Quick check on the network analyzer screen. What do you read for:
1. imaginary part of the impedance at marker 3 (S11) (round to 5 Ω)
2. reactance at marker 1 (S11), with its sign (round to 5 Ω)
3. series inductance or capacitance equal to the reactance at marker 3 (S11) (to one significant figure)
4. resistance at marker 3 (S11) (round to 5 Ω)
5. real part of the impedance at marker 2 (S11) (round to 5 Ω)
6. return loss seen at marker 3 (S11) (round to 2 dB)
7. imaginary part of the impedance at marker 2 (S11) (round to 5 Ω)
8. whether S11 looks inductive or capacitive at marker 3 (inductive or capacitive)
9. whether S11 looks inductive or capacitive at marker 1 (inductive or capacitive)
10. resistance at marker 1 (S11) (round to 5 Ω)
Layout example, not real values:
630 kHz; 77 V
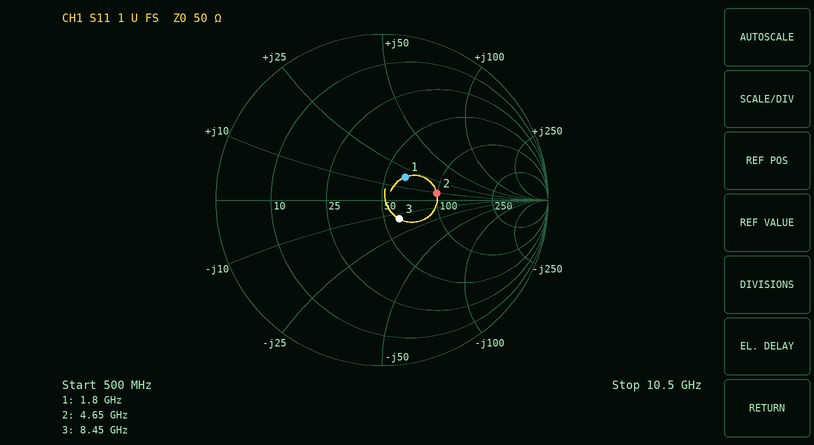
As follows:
-15 Ω; +20 Ω; 1 pF; 60 Ω; 100 Ω; 16 dB; +10 Ω; capacitive; inductive; 65 Ω
